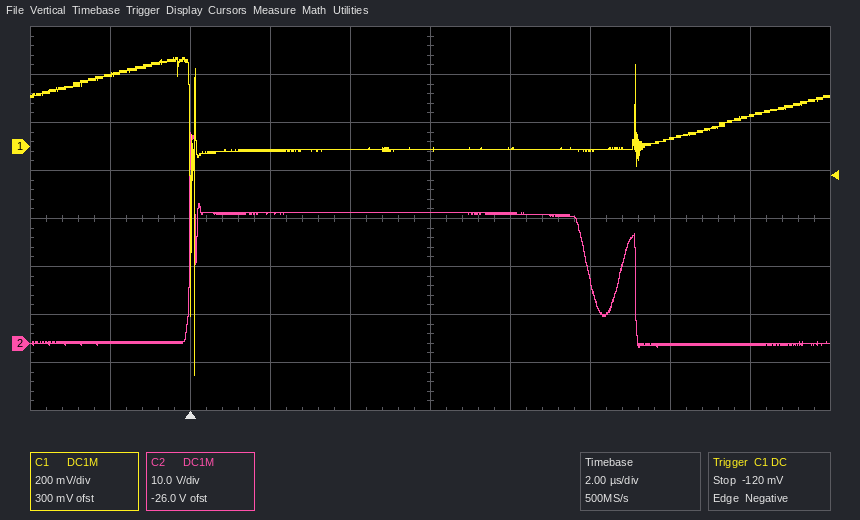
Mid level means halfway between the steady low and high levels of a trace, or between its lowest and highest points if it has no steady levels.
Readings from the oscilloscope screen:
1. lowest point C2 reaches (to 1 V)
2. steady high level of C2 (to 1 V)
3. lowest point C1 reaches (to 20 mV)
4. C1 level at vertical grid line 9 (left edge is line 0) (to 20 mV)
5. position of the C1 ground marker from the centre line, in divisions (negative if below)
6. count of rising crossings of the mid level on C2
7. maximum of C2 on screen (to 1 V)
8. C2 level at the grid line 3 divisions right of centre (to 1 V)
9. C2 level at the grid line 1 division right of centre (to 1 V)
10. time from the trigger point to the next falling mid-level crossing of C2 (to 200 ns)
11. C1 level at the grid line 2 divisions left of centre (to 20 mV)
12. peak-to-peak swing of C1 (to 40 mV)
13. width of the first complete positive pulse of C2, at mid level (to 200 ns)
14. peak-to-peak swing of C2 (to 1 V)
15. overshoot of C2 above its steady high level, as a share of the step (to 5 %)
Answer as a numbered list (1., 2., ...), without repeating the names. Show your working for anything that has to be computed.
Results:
1. -1 V
2. 27 V
3. -960 mV
4. 120 mV
5. +1.5 div
6. 2
7. 44 V
8. 0 V
9. 27 V
10. 10.0 µs
11. -20 mV
12. 1.32 V
13. 10.0 µs
14. 44 V − (-1 V) = 45 V
15. 60 %
